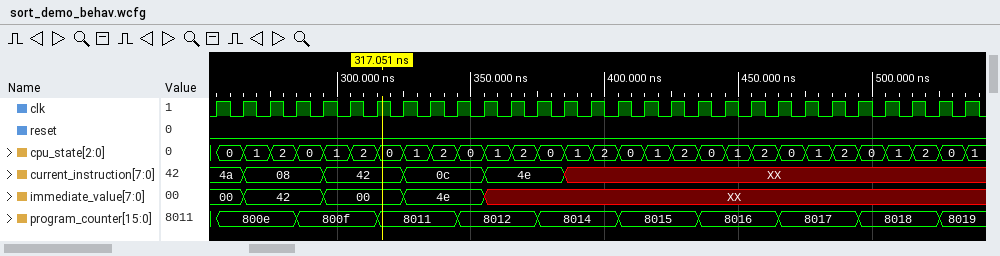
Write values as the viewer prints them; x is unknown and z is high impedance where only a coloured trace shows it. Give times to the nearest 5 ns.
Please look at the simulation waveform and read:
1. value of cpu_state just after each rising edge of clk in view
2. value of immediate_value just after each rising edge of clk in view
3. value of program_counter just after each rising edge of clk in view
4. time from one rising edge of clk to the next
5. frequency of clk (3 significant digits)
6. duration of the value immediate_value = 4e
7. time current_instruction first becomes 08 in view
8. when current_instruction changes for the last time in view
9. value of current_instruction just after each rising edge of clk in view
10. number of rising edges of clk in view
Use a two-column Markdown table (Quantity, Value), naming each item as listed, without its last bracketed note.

| Quantity | Value |
|---|---|
| value of cpu_state just after each rising edge of clk in view | 0, 1, 2, 0, 1, 2, 0, 1, 2, 0, 1, 2, 0, 1, 2, 0, 1, 2, 0, 1, 2, 0, 1, 2, 0, 1, 2, 0, 1 |
| value of immediate_value just after each rising edge of clk in view | 00, 42, 42, 42, 00, 00, 00, 4e, 4e, 4e, XX, XX, XX, XX, XX, XX, XX, XX, XX, XX, XX, XX, XX, XX, XX, XX, XX, XX, XX |
| value of program_counter just after each rising edge of clk in view | 800e, 800e, 800e, 800f, 800f, 800f, 8011, 8011, 8011, 8012, 8012, 8012, 8014, 8014, 8014, 8015, 8015, 8015, 8016, 8016, 8016, 8017, 8017, 8017, 8018, 8018, 8018, 8019, 8019 |
| time from one rising edge of clk to the next | 10 ns |
| frequency of clk | 100 MHz |
| duration of the value immediate_value = 4e | 30 ns |
| time current_instruction first becomes 08 in view | 265 ns |
| when current_instruction changes for the last time in view | 385 ns |
| value of current_instruction just after each rising edge of clk in view | 4a, 08, 08, 08, 42, 42, 42, 0c, 0c, 0c, 4e, 4e, 4e, XX, XX, XX, XX, XX, XX, XX, XX, XX, XX, XX, XX, XX, XX, XX, XX |
| number of rising edges of clk in view | 29 |
